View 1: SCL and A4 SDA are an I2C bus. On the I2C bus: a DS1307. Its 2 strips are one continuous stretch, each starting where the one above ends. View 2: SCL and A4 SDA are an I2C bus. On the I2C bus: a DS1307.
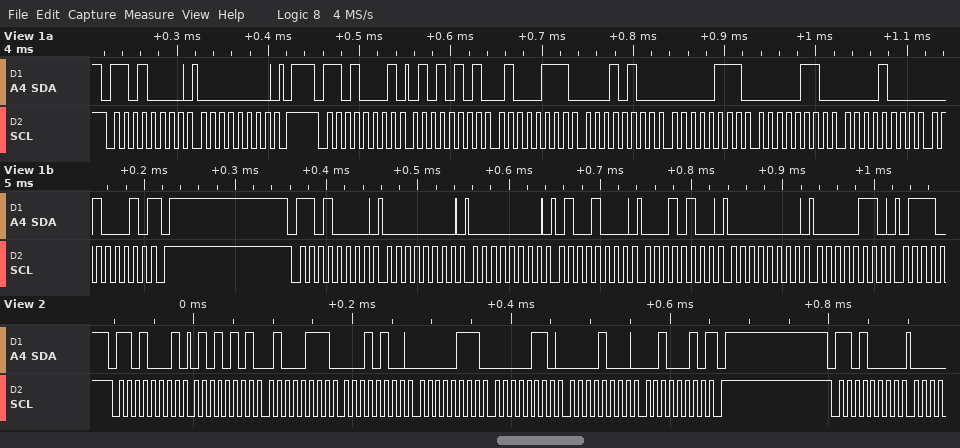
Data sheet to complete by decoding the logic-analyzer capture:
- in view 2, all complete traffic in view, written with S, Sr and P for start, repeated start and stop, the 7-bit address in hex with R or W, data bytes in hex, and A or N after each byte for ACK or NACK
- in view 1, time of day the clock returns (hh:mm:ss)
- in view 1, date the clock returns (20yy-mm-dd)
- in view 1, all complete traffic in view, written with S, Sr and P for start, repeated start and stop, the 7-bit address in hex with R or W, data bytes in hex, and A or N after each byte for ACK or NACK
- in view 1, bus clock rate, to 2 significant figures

S 68R A 55 A 47 A 14 A 07 A 06 A 08 A 22 N P S 68W A
14:47:55
2022-08-06
S 68W A 00 A P S 68R A 55 A 47 A 14 A 07 A 06 A 08 A 22 N P S 68W A 00 A 00 A 48 A 14 A 00 A 06 A
100 kHz
